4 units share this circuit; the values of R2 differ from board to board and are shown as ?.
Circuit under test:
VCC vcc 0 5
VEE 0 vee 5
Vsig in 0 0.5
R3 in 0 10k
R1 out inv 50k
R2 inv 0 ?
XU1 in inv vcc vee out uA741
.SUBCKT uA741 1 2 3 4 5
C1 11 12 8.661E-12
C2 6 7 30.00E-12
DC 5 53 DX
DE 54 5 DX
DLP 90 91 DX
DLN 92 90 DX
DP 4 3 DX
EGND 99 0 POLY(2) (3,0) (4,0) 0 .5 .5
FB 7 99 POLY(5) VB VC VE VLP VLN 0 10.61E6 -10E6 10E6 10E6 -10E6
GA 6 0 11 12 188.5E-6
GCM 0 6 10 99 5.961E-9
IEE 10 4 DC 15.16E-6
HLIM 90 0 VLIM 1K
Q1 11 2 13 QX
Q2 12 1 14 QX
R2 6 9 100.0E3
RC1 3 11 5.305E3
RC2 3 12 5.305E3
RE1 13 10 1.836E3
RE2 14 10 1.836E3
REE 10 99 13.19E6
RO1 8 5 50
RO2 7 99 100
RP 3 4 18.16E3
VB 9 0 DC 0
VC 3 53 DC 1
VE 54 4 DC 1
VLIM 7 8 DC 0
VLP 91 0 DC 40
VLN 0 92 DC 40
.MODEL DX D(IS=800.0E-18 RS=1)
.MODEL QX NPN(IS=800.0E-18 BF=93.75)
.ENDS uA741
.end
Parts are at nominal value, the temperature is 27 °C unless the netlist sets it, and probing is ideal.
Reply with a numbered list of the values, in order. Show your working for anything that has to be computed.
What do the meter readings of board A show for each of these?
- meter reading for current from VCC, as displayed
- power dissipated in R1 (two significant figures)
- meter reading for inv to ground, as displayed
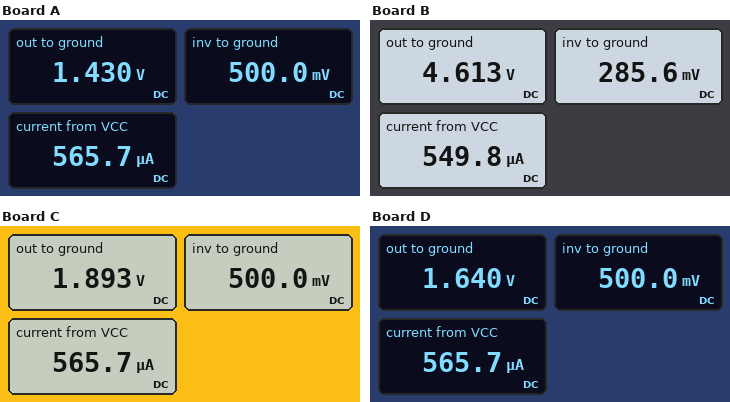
1. 565.7 µA
2. (1.43 V - 500 mV)^2 / 50 kΩ = 17 µW
3. 500.0 mV
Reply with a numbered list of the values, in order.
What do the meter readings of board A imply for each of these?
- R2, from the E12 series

1. 27 kΩ
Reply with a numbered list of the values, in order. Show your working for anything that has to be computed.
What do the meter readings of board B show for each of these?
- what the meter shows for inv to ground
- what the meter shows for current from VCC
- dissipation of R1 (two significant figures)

1. 285.6 mV
2. 549.8 µA
3. (4.613 V - 285.6 mV)^2 / 50 kΩ = 370 µW
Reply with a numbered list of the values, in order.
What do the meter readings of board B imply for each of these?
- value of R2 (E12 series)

1. 3.3 kΩ
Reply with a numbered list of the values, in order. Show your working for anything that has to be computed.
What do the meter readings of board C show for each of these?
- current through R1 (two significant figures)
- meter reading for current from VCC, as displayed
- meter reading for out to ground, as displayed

1. (1.893 V - 500 mV) / 50 kΩ = 28 µA
2. 565.7 µA
3. 1.893 V
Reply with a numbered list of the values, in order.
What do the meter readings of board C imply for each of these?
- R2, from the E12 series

1. 18 kΩ
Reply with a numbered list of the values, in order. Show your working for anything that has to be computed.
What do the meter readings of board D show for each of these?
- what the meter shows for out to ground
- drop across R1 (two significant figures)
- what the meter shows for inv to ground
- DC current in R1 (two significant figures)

1. 1.640 V
2. 1.64 V - 500 mV = 1.1 V
3. 500.0 mV
4. (1.64 V - 500 mV) / 50 kΩ = 23 µA
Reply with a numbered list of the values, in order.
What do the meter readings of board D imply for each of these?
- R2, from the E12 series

1. 22 kΩ
